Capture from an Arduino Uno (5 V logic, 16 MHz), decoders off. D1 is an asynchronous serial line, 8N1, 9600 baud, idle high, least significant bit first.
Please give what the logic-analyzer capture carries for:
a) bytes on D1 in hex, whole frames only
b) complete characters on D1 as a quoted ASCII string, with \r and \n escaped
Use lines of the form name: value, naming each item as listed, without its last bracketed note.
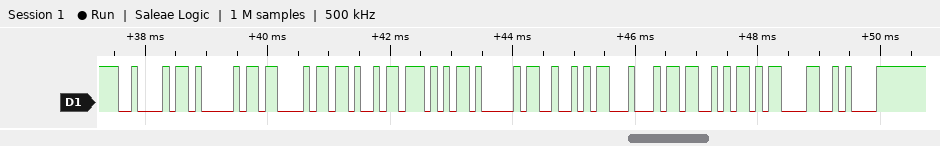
bytes on D1 in hex, whole frames only: 0x42 0x41 0x43 0x4B 0x57 0x41 0x52 0x44 0x53 0x0D 0x0A
complete characters on D1 as a quoted ASCII string, with \r and \n escaped: "BACKWARDS\r\n"
